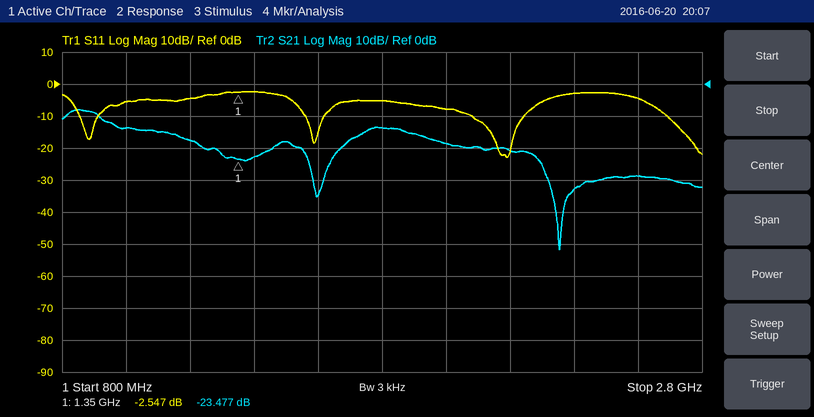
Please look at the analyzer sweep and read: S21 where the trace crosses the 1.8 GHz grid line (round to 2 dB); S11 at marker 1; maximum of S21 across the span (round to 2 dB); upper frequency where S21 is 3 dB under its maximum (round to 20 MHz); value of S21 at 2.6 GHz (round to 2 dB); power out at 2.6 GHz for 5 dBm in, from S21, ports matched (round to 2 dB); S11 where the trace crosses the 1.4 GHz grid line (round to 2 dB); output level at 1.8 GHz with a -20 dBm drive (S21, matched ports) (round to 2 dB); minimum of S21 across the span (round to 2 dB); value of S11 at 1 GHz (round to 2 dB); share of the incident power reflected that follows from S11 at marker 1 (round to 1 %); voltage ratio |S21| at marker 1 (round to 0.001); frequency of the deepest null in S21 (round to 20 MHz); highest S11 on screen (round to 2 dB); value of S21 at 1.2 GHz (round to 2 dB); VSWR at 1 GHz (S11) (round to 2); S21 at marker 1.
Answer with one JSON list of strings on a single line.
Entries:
["-14 dB", "-2.547 dB", "-8 dB", "920 MHz", "-28 dB", "-24 dBm", "-2 dB", "-34 dBm", "-52 dB", "-6 dB", "56 %", "0.067", "2.36 GHz", "-2 dB", "-18 dB", "4", "-23.477 dB"]
